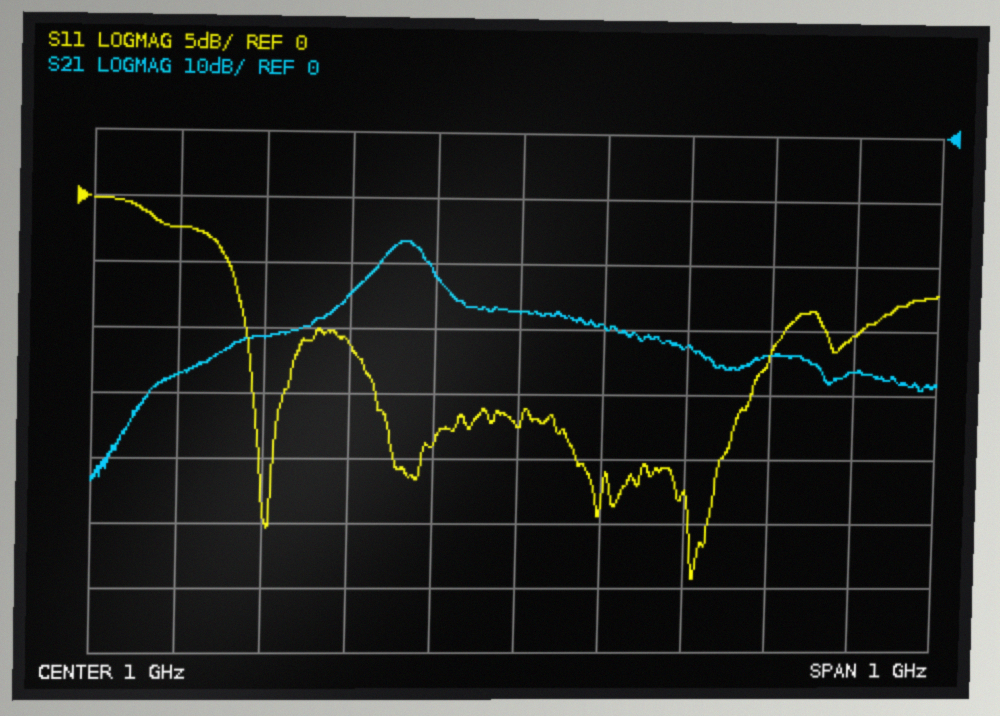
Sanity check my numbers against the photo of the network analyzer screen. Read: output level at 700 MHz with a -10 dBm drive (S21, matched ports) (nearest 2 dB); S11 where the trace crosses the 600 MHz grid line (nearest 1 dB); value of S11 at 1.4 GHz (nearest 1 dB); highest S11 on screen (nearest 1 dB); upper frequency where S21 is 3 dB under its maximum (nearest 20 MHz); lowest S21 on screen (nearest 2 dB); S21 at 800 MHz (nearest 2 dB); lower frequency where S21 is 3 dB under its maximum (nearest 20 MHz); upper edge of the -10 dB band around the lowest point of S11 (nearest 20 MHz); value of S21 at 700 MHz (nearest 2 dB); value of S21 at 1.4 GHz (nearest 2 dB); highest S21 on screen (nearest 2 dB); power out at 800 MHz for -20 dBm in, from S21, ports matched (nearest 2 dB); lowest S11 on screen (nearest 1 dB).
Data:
-42 dBm
-2 dB
-10 dB
0 dB
880 MHz
-54 dB
-24 dB
840 MHz
1.32 GHz
-32 dB
-36 dB
-16 dB
-44 dBm
-29 dB
